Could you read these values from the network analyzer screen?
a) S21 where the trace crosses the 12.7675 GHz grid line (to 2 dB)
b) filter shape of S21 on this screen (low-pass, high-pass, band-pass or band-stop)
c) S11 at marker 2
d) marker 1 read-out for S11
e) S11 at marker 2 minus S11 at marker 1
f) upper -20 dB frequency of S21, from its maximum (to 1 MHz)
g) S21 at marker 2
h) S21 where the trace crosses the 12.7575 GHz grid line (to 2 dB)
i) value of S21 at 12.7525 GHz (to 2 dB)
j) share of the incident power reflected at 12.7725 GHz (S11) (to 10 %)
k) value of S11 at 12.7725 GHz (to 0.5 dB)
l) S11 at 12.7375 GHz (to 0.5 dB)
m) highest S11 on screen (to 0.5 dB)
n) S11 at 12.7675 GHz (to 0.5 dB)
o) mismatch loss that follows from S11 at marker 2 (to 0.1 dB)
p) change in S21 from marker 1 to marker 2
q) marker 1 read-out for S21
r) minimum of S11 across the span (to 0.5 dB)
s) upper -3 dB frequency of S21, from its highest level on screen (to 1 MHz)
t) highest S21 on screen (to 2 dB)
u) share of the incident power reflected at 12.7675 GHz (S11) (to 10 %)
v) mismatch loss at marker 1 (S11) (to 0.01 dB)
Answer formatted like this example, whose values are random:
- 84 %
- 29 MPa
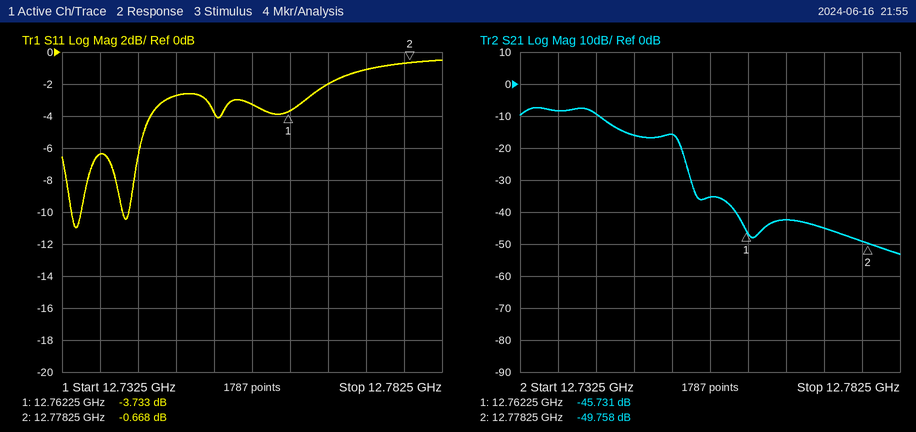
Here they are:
- -42 dB
- low-pass
- -0.668 dB
- -3.733 dB
- 3.065 dB
- 12.755 GHz
- -49.758 dB
- -36 dB
- -16 dB
- 80 %
- -1.0 dB
- -6.5 dB
- -0.5 dB
- -2.0 dB
- 8.5 dB
- -4.027 dB
- -45.731 dB
- -11.0 dB
- 12.743 GHz
- -8 dB
- 60 %
- 2.39 dB
